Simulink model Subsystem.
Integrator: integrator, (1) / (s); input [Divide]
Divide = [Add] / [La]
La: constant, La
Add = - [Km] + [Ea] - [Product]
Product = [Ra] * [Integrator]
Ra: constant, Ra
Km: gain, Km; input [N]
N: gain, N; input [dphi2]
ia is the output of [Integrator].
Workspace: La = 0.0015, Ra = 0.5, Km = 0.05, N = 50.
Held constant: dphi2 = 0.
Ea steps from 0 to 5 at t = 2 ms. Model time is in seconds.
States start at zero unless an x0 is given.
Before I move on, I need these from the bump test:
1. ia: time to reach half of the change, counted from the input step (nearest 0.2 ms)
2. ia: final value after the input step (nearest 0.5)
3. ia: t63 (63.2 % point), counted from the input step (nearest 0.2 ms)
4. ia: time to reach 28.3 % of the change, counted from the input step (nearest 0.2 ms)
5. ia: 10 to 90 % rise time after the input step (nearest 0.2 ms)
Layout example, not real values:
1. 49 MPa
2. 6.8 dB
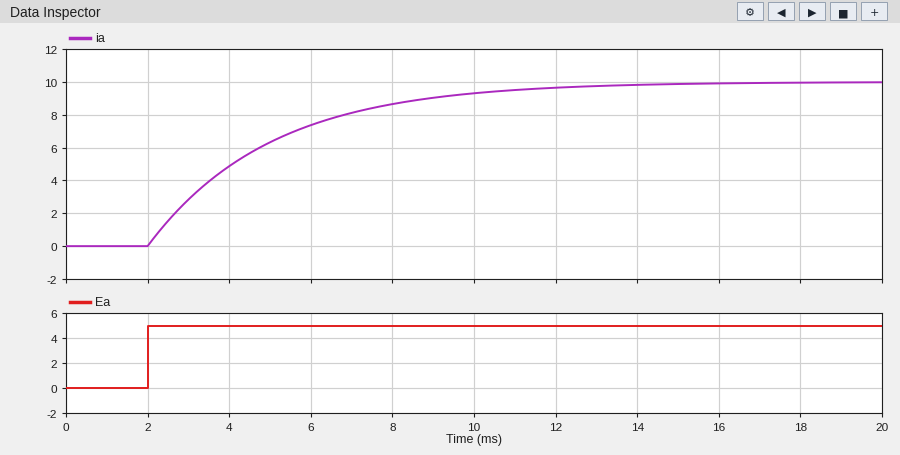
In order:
1. 2.0 ms
2. 10.0
3. 3.0 ms
4. 1.0 ms
5. 6.6 ms
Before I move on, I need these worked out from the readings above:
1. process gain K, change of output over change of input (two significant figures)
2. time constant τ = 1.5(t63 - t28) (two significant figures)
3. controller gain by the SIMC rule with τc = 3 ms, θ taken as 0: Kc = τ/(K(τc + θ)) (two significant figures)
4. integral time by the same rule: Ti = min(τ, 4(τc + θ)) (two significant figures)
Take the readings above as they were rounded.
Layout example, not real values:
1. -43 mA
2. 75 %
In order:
1. 2.0
2. 3.0 ms
3. 0.50
4. 3.0 ms
